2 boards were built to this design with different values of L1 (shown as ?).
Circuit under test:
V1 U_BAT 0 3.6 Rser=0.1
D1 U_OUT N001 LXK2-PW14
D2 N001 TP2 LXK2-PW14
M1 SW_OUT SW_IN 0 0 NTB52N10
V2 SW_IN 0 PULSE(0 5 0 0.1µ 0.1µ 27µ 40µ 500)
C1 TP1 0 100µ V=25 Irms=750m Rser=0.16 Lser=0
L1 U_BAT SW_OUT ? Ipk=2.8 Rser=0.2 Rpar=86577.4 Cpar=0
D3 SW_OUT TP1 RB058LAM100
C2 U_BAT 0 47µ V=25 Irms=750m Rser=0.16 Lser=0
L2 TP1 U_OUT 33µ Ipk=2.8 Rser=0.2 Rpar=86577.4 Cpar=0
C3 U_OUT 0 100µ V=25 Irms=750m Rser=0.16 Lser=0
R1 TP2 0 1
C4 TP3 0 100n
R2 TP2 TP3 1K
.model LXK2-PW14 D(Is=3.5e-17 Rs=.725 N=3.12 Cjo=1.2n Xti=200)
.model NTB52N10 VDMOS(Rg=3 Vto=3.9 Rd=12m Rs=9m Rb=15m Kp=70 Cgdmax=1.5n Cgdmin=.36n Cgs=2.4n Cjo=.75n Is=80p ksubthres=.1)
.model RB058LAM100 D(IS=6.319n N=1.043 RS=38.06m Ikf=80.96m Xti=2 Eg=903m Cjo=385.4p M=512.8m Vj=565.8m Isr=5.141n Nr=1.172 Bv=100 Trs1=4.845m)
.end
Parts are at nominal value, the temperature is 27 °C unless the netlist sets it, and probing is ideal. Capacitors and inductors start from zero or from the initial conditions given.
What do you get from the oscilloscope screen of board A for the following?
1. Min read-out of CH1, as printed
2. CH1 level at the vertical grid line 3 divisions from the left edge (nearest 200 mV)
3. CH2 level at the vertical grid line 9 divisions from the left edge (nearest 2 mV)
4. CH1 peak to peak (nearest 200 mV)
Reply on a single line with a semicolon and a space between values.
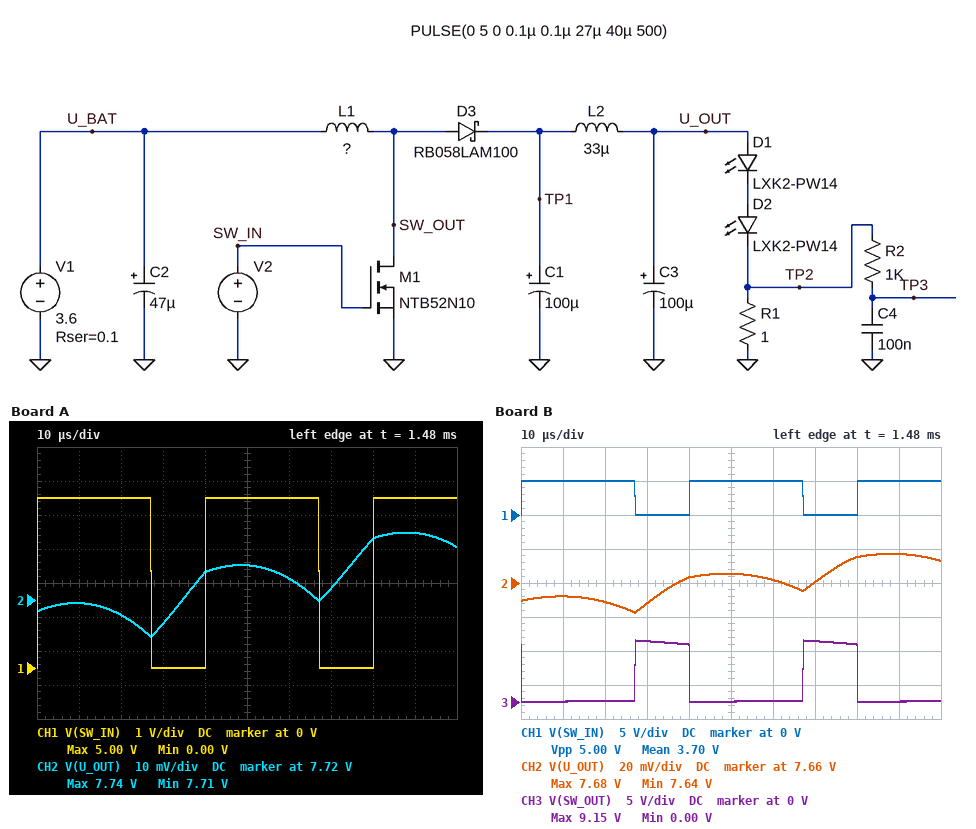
0.00 V; 0 V; 7.740 V; 5.0 V
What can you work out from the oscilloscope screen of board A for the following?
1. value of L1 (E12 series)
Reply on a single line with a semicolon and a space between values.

39 µH
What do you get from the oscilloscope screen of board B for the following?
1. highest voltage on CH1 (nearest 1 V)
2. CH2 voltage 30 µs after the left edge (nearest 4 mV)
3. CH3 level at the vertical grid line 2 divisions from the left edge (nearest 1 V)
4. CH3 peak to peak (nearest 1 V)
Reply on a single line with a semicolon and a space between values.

5 V; 7.648 V; 0 V; 9 V
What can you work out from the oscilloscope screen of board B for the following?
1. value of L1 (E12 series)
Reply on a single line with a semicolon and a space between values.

22 µH
